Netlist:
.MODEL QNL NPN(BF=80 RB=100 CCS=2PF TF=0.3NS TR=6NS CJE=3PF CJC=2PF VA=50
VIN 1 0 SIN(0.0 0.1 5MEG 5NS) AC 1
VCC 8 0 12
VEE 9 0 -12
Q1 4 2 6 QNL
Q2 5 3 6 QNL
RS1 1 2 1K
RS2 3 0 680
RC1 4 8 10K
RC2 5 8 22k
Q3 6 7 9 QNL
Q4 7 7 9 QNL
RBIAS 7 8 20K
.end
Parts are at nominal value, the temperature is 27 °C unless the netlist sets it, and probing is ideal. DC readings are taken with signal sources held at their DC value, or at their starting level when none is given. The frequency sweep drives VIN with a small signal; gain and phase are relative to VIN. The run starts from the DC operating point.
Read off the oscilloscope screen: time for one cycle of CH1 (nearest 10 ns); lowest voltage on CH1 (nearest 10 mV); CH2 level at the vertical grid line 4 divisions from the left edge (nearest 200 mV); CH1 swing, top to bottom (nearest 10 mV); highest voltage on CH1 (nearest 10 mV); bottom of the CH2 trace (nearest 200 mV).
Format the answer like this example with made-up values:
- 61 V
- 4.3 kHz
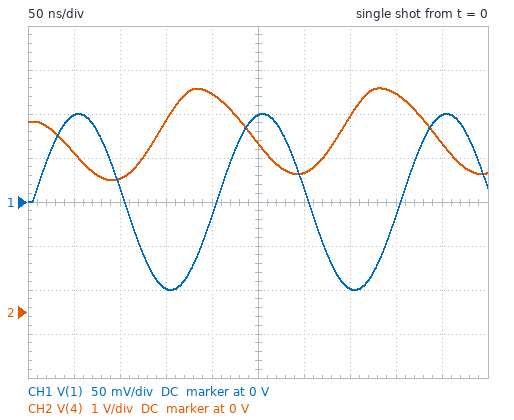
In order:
- 200 ns
- -100 mV
- 5.0 V
- 200 mV
- 100 mV
- 3.0 V
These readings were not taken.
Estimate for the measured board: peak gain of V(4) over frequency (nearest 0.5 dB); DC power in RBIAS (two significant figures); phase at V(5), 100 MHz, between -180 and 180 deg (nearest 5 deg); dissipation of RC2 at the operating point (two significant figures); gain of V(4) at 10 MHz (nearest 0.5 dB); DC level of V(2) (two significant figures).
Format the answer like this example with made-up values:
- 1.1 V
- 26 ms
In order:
- 22.0 dB
- 27 mW
- -85 deg
- 7.3 mW
- 14.0 dB
- -8.8 mV
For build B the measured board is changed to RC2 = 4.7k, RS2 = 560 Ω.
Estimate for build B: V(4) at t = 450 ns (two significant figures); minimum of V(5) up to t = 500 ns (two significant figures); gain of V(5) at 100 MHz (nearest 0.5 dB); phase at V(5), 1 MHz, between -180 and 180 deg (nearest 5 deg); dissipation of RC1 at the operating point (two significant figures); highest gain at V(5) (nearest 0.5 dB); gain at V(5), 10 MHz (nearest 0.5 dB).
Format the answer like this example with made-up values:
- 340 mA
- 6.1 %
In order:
- 5.7 V
- 7.6 V
- -7.5 dB
- -40 deg
- 3.9 mW
- 33.0 dB
- 16.5 dB
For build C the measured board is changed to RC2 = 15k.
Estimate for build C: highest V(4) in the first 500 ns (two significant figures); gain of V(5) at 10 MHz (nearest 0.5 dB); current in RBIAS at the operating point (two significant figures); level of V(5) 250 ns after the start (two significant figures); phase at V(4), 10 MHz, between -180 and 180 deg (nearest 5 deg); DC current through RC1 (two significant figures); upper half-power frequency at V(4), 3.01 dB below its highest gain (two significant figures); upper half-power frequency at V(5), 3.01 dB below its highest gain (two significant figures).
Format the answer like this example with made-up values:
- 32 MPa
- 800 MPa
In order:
- 6.2 V
- 16.0 dB
- 1.2 mA
- 2.1 V
- 95 deg
- 670 µA
- 580 kHz
- 570 kHz
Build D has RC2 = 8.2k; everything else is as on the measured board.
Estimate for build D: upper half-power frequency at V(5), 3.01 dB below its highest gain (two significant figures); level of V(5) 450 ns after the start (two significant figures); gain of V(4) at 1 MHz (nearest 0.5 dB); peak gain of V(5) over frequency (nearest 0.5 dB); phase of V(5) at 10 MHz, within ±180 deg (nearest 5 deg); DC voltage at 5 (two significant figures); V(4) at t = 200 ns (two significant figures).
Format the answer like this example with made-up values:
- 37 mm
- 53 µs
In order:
- 840 kHz
- 6.3 V
- 35.5 dB
- 37.5 dB
- -90 deg
- 6.2 V
- 6.4 V
